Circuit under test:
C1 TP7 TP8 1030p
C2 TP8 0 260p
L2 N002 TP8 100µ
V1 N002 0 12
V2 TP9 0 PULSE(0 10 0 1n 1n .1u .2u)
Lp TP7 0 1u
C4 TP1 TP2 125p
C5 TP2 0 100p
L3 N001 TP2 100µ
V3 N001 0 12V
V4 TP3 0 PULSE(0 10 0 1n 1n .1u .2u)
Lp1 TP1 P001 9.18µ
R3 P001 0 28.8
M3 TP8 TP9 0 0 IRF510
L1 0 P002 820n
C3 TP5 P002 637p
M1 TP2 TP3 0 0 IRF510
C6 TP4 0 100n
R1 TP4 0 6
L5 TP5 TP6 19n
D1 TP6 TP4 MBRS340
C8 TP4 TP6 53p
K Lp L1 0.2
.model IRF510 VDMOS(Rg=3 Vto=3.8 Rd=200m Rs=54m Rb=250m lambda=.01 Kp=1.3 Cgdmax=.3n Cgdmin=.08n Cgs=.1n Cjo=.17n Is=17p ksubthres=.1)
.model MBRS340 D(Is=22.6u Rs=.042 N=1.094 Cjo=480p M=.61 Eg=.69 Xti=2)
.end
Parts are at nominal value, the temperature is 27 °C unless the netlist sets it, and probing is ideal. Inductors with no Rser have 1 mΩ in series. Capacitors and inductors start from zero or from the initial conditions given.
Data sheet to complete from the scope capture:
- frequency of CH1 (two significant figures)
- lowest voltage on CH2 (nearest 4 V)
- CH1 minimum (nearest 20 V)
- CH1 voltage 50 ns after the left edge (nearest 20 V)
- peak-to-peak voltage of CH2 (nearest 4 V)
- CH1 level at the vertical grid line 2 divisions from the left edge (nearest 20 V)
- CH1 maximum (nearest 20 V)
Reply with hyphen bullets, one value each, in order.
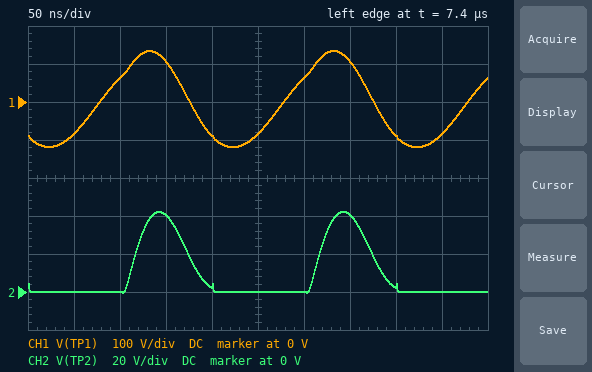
- 5.0 MHz
- 0 V
- -120 V
- -80 V
- 44 V
- 60 V
- 140 V
